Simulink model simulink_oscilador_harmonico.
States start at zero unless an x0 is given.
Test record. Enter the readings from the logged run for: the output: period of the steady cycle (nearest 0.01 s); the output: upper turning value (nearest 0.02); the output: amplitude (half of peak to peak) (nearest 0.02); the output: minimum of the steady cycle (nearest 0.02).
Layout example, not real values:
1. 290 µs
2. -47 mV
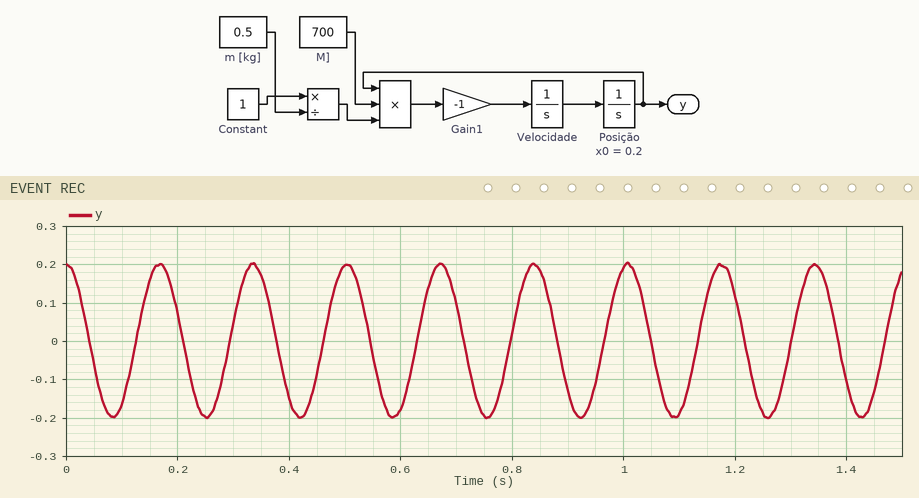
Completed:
1. 0.17 s
2. 0.20
3. 0.20
4. -0.20
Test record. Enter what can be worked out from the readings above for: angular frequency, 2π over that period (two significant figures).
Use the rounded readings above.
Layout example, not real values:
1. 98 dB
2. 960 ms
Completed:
1. 37 rad/s
